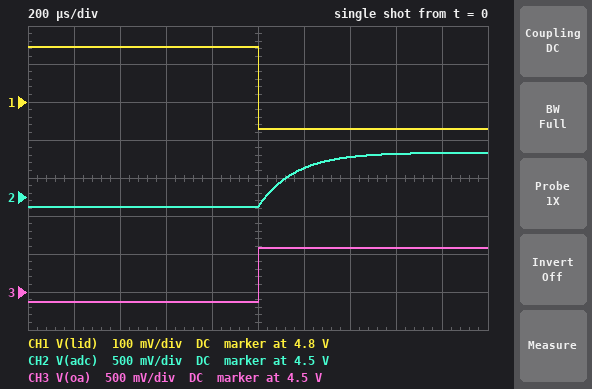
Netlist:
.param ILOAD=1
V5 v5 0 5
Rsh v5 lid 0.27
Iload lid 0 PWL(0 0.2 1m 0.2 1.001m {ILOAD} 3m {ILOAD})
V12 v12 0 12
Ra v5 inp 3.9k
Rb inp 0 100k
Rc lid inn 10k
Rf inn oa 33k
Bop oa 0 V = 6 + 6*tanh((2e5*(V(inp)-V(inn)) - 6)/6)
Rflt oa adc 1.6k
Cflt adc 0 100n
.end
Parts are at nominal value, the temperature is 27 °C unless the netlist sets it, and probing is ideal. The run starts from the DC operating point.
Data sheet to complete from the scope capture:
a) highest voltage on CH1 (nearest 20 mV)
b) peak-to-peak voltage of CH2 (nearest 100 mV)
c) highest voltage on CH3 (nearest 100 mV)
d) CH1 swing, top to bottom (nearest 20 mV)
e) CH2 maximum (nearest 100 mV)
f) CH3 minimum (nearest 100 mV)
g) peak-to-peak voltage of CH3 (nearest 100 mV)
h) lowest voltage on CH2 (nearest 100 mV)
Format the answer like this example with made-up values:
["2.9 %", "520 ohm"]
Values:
["4.94 V", "700 mV", "5.1 V", "220 mV", "5.1 V", "4.4 V", "700 mV", "4.4 V"]
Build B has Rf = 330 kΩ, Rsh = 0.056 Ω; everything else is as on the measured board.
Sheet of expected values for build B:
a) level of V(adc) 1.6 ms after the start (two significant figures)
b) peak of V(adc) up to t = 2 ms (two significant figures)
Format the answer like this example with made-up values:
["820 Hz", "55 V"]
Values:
["460 mV", "470 mV"]
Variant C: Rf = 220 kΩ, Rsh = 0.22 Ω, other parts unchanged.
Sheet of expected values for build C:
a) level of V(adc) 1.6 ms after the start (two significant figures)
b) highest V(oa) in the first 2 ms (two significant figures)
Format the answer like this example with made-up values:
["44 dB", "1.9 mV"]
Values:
["5.4 V", "5.5 V"]
